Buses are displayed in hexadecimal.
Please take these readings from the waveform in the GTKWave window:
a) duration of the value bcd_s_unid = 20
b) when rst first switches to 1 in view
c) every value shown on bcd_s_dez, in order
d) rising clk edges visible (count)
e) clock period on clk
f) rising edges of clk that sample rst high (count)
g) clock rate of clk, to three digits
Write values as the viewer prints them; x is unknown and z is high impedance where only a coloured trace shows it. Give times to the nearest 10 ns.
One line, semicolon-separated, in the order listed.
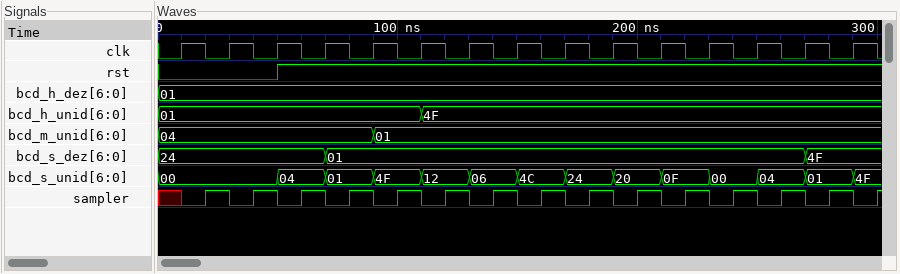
20 ns; 50 ns; 24, 01, 4F; 15; 20 ns; 12; 50.0 MHz
